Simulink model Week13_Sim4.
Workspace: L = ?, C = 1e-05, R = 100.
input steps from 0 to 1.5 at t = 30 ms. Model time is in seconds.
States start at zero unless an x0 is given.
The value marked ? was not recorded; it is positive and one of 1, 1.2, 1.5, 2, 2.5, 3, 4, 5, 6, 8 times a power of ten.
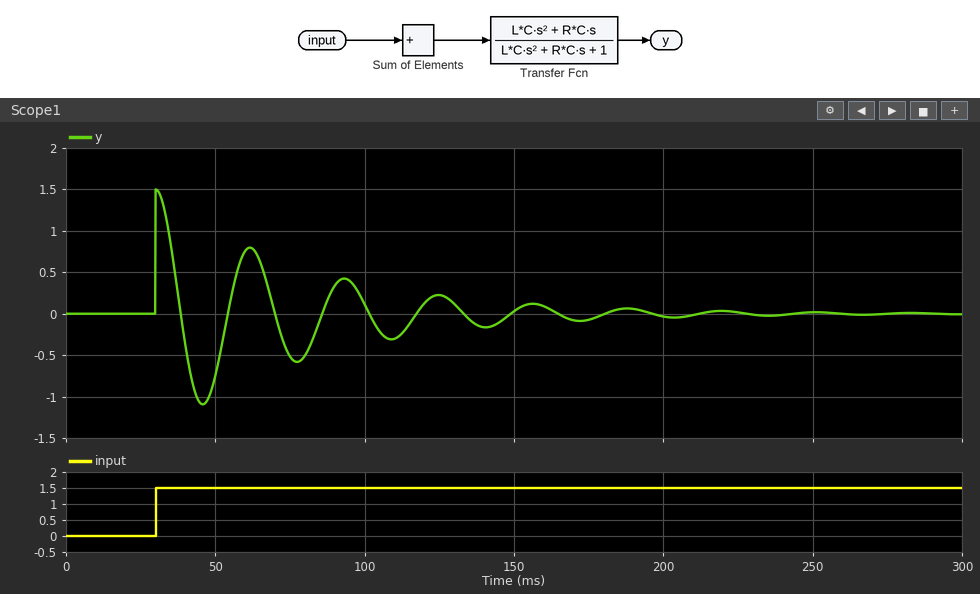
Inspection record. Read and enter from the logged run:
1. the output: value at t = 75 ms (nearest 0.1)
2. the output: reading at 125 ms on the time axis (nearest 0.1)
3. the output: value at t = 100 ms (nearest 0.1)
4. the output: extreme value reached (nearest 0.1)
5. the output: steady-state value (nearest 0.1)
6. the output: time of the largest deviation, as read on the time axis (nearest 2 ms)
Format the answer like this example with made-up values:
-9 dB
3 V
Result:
-0.5
0.2
0.1
1.5
0.0
30 ms
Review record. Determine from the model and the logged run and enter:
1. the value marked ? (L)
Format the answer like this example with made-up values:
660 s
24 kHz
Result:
2.5
